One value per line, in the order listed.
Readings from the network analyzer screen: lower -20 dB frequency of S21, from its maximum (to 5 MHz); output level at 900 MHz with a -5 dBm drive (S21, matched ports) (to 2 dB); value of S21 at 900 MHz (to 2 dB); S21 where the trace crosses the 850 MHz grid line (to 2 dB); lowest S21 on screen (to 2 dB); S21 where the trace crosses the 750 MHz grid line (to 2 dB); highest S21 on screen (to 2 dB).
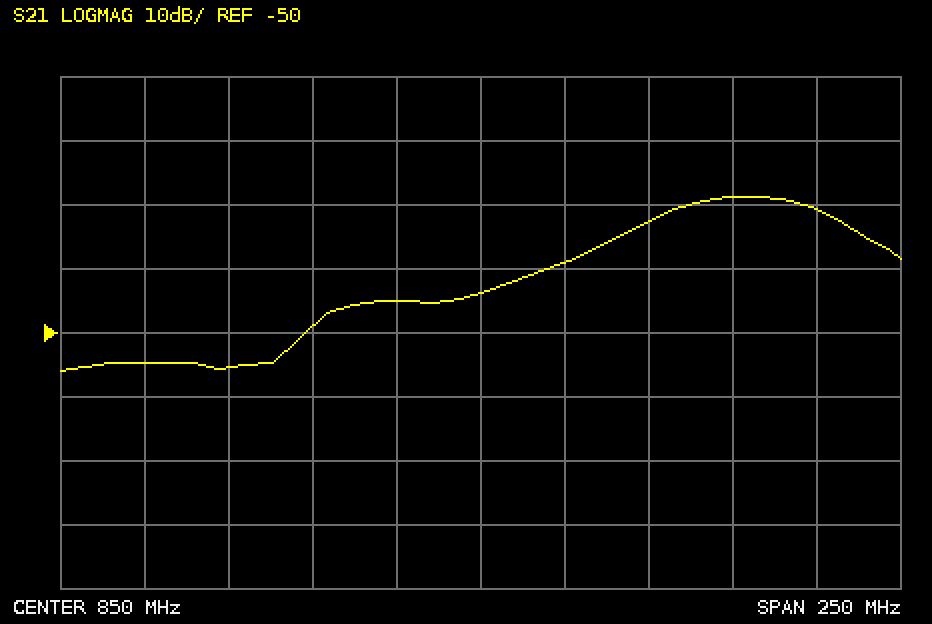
800 MHz
-38 dBm
-32 dB
-44 dB
-56 dB
-54 dB
-28 dB
